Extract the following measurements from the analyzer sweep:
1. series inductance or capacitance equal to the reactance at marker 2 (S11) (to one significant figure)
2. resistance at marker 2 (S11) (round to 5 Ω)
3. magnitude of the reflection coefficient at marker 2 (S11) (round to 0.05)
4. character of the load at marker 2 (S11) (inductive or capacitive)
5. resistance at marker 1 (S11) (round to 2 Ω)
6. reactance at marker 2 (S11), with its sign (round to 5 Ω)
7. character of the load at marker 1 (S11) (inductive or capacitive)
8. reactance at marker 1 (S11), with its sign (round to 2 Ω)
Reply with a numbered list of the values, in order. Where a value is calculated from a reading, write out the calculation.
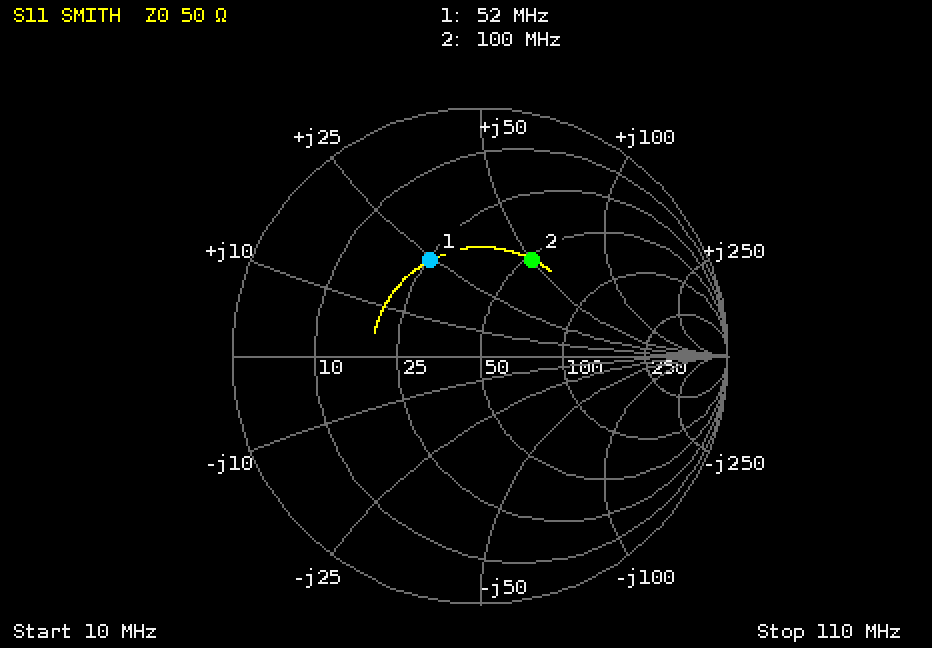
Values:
1. L = 50 Ω/(2π × 100 MHz) ≈ 80 nH
2. 50 Ω
3. 0.45
4. inductive
5. 26 Ω
6. +50 Ω
7. inductive
8. +24 Ω
